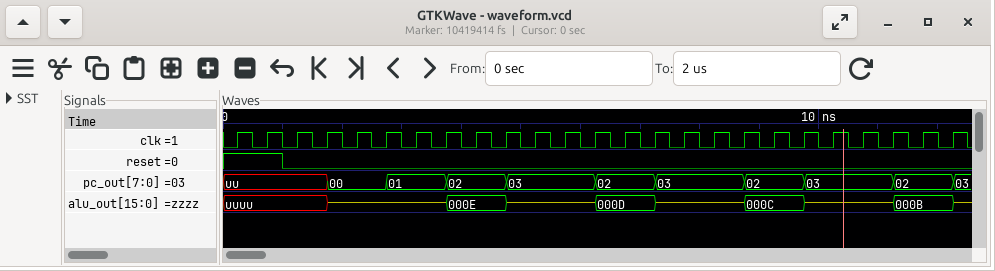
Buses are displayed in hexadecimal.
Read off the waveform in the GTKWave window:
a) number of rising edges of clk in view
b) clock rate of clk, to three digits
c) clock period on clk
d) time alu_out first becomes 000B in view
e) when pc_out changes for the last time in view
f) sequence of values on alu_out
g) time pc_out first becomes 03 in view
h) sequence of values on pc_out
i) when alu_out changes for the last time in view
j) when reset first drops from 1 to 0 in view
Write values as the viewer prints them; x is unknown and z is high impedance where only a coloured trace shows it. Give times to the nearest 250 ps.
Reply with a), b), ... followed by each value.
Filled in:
a) 25
b) 2.00 GHz
c) 500 ps
d) 11250 ps
e) 12250 ps
f) uuuu, z, 000E, z, 000D, z, 000C, z, 000B, z
g) 4750 ps
h) uu, 00, 01, 02, 03, 02, 03, 02, 03, 02, 03
i) 12250 ps
j) 1000 ps
